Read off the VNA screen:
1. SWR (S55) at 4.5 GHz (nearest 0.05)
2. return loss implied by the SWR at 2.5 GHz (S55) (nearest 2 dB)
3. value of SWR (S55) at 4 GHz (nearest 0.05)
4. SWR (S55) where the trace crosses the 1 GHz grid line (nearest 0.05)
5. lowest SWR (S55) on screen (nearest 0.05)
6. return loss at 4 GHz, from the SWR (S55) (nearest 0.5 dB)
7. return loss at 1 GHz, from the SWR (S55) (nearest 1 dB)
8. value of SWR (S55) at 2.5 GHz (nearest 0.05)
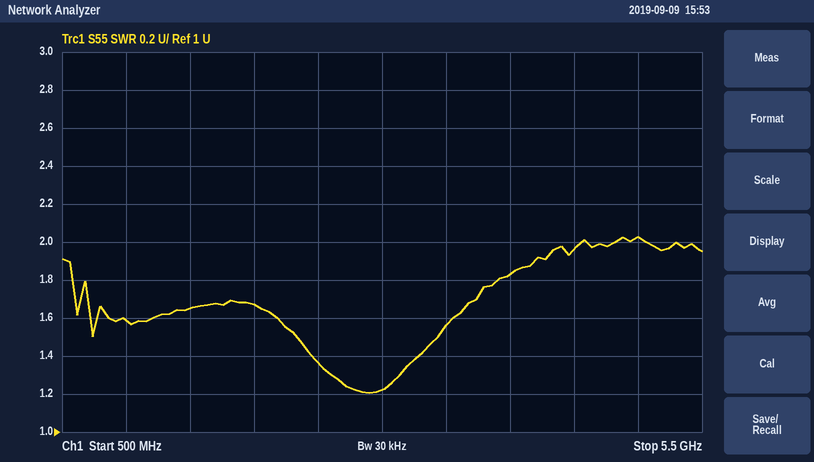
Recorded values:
1.95
16 dB
1.85
1.60
1.20
10.5 dB
13 dB
1.35
